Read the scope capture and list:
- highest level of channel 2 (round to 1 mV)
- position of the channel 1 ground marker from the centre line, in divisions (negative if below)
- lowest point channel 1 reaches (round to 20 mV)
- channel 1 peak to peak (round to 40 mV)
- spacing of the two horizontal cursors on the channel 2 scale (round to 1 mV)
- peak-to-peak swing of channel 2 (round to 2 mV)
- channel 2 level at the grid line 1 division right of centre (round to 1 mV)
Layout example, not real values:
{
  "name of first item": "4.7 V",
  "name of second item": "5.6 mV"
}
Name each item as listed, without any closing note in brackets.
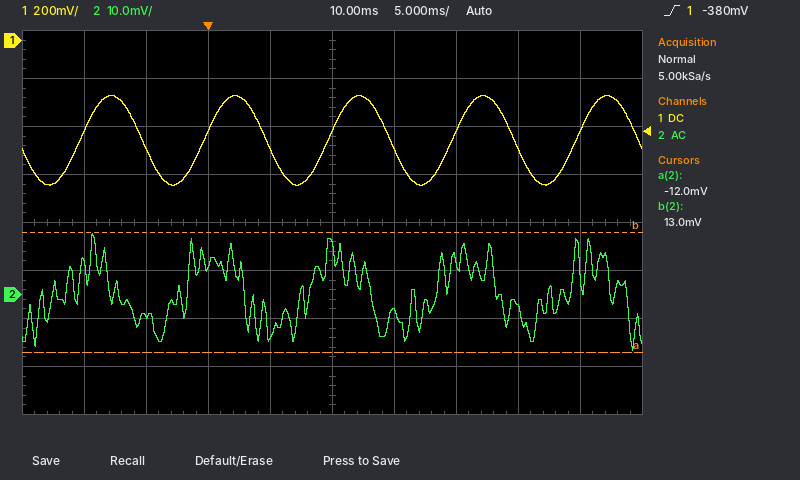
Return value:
{
  "highest level of channel 2": "13 mV",
  "position of the channel 1 ground marker from the centre line, in divisions": "+3.8 div",
  "lowest point channel 1 reaches": "-600 mV",
  "channel 1 peak to peak": "360 mV",
  "spacing of the two horizontal cursors on the channel 2 scale": "25 mV",
  "peak-to-peak swing of channel 2": "24 mV",
  "channel 2 level at the grid line 1 division right of centre": "-4 mV"
}
